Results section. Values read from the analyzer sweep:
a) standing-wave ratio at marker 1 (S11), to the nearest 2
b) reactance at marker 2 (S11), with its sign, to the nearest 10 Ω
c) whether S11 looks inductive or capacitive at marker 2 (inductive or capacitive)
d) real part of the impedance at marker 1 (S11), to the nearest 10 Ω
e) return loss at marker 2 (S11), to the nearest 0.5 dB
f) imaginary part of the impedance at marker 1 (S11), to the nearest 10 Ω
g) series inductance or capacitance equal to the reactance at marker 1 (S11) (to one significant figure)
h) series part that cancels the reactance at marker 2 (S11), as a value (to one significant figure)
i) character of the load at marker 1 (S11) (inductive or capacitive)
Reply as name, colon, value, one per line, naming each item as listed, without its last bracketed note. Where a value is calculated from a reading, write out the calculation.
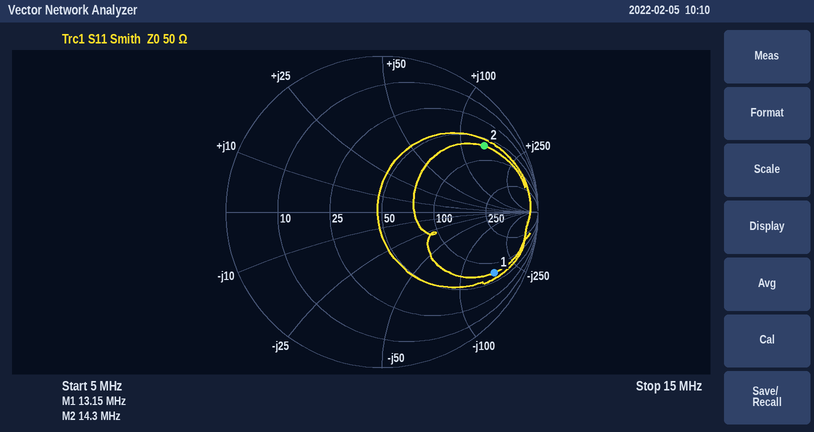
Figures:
standing-wave ratio at marker 1 (S11), to the nearest 2: 10
reactance at marker 2 (S11), with its sign, to the nearest 10 Ω: +140 Ω
whether S11 looks inductive or capacitive at marker 2: inductive
real part of the impedance at marker 1 (S11), to the nearest 10 Ω: 70 Ω
return loss at marker 2 (S11), to the nearest 0.5 dB: 2.0 dB
imaginary part of the impedance at marker 1 (S11), to the nearest 10 Ω: -170 Ω
series inductance or capacitance equal to the reactance at marker 1 (S11): C = 1/(2π × 13.15 MHz × 170 Ω) ≈ 71.2 pF, so 70 pF to one significant figure
series part that cancels the reactance at marker 2 (S11), as a value: C = 1/(2π × 14.3 MHz × 140 Ω) ≈ 80 pF
character of the load at marker 1 (S11): capacitive
